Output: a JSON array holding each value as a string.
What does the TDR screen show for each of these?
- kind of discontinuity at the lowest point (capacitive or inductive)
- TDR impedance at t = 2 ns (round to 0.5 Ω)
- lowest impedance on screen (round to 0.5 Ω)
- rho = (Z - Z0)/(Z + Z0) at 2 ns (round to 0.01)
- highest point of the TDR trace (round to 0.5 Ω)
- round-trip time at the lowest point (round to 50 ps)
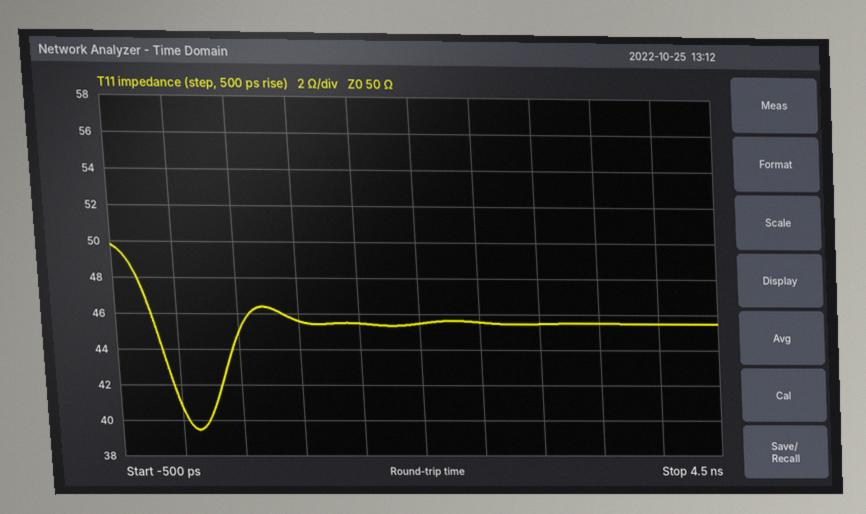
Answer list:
["capacitive", "45.5 Ω", "39.5 Ω", "-0.05", "50.0 Ω", "150 ps"]
